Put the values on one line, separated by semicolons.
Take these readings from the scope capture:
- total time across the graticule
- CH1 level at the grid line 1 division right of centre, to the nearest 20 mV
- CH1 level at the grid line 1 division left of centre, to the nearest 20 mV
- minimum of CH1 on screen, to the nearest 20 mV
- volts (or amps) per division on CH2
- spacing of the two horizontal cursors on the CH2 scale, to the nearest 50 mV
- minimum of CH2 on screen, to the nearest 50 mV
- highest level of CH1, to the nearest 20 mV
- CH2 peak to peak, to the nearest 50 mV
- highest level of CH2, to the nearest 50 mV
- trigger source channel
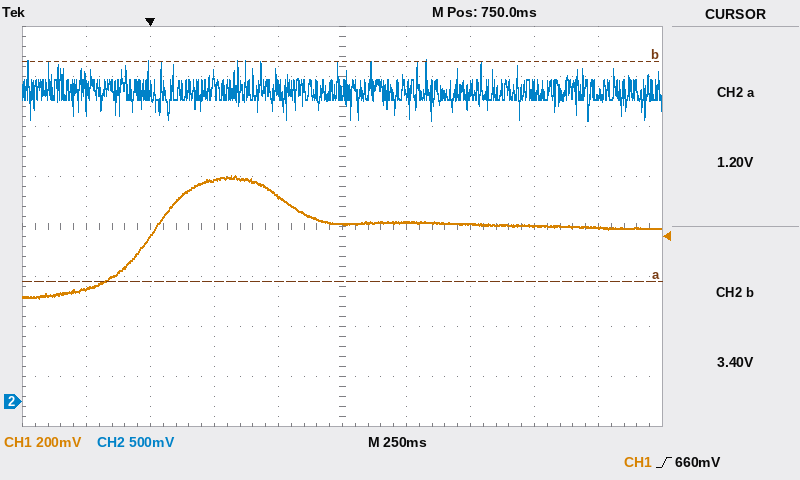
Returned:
2.5 s; 720 mV; 820 mV; 420 mV; 500 mV; 2.20 V; 2.80 V; 900 mV; 600 mV; 3.40 V; CH1
